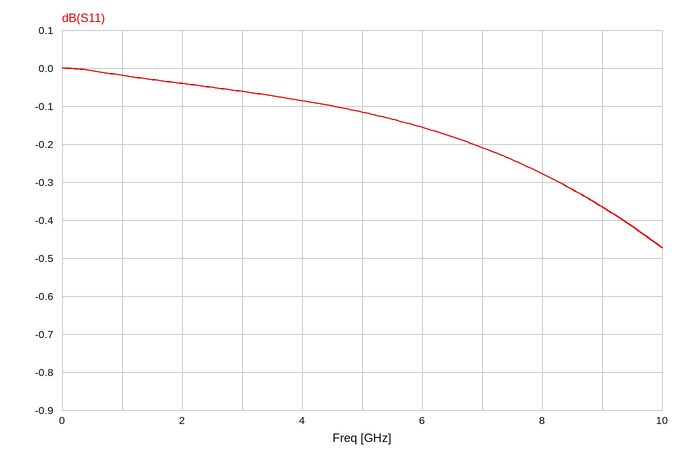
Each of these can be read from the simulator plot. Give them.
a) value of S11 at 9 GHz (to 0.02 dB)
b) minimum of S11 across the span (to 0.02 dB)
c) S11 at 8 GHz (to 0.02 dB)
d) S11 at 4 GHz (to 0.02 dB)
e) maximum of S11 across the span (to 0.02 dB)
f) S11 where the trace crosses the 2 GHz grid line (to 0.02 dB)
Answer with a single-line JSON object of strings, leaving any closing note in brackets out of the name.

{"value of S11 at 9 GHz": "-0.36 dB", "minimum of S11 across the span": "-0.48 dB", "S11 at 8 GHz": "-0.28 dB", "S11 at 4 GHz": "-0.08 dB", "maximum of S11 across the span": "0.00 dB", "S11 where the trace crosses the 2 GHz grid line": "-0.04 dB"}
